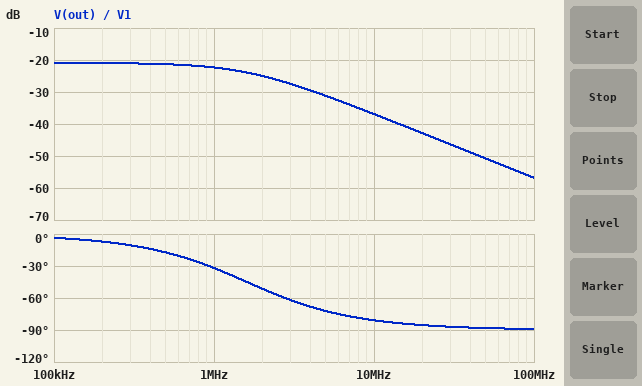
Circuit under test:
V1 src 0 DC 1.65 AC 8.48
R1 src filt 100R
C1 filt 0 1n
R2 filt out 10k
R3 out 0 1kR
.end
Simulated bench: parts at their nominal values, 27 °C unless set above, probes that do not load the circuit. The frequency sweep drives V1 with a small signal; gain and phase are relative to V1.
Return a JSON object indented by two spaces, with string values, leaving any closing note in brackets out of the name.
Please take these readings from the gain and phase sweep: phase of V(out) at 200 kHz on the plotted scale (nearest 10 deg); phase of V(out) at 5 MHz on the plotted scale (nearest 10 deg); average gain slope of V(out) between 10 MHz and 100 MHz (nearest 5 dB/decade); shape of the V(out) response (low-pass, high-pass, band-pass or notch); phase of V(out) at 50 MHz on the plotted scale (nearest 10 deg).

{
  "phase of V(out) at 200 kHz on the plotted scale": "-10 deg",
  "phase of V(out) at 5 MHz on the plotted scale": "-70 deg",
  "average gain slope of V(out) between 10 MHz and 100 MHz": "-20 dB/decade",
  "shape of the V(out) response": "low-pass",
  "phase of V(out) at 50 MHz on the plotted scale": "-90 deg"
}
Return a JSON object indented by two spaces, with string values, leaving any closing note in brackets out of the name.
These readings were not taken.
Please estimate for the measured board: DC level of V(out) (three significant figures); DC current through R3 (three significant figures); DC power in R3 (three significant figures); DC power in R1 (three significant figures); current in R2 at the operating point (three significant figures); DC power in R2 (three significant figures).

{
  "DC level of V(out)": "149 mV",
  "DC current through R3": "149 µA",
  "DC power in R3": "22.1 µW",
  "DC power in R1": "2.21 µW",
  "current in R2 at the operating point": "149 µA",
  "DC power in R2": "221 µW"
}
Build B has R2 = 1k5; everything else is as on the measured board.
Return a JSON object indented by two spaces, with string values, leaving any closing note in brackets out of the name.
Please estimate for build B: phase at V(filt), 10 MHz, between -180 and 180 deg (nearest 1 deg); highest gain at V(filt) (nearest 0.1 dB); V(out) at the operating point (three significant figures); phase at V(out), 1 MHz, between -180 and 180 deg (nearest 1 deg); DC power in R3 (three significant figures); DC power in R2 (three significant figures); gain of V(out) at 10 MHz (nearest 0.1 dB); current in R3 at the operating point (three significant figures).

{
  "phase at V(filt), 10 MHz, between -180 and 180 deg": "-81 deg",
  "highest gain at V(filt)": "-0.3 dB",
  "V(out) at the operating point": "635 mV",
  "phase at V(out), 1 MHz, between -180 and 180 deg": "-31 deg",
  "DC power in R3": "403 µW",
  "DC power in R2": "604 µW",
  "gain of V(out) at 10 MHz": "-24.0 dB",
  "current in R3 at the operating point": "635 µA"
}
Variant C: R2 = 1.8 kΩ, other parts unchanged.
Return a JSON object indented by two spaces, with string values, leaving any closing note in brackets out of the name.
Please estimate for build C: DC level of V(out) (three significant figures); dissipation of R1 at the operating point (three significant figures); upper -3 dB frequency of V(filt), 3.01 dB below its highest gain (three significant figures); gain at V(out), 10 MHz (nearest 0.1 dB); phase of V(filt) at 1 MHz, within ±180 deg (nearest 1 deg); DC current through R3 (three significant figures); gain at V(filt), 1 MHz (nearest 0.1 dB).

{
  "DC level of V(out)": "569 mV",
  "dissipation of R1 at the operating point": "32.4 µW",
  "upper -3 dB frequency of V(filt), 3.01 dB below its highest gain": "1.65 MHz",
  "gain at V(out), 10 MHz": "-25.0 dB",
  "phase of V(filt) at 1 MHz, within ±180 deg": "-31 deg",
  "DC current through R3": "569 µA",
  "gain at V(filt), 1 MHz": "-1.7 dB"
}
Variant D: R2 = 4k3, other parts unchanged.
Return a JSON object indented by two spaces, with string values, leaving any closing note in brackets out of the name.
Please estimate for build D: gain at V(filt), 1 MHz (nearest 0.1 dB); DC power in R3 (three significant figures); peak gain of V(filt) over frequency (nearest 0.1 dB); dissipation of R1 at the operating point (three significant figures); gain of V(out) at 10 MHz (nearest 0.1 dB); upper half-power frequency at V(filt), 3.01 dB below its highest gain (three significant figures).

{
  "gain at V(filt), 1 MHz": "-1.6 dB",
  "DC power in R3": "93.4 µW",
  "peak gain of V(filt) over frequency": "-0.2 dB",
  "dissipation of R1 at the operating point": "9.34 µW",
  "gain of V(out) at 10 MHz": "-30.6 dB",
  "upper half-power frequency at V(filt), 3.01 dB below its highest gain": "1.62 MHz"
}
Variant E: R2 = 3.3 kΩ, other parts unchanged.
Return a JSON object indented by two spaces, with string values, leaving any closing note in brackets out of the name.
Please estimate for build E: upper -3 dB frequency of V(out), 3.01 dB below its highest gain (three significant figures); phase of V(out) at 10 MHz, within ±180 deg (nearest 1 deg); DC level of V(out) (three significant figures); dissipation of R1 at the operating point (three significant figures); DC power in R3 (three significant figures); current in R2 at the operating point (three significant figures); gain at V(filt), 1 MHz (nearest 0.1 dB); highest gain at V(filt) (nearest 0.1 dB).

{
  "upper -3 dB frequency of V(out), 3.01 dB below its highest gain": "1.63 MHz",
  "phase of V(out) at 10 MHz, within ±180 deg": "-81 deg",
  "DC level of V(out)": "375 mV",
  "dissipation of R1 at the operating point": "14.1 µW",
  "DC power in R3": "141 µW",
  "current in R2 at the operating point": "375 µA",
  "gain at V(filt), 1 MHz": "-1.6 dB",
  "highest gain at V(filt)": "-0.2 dB"
}
